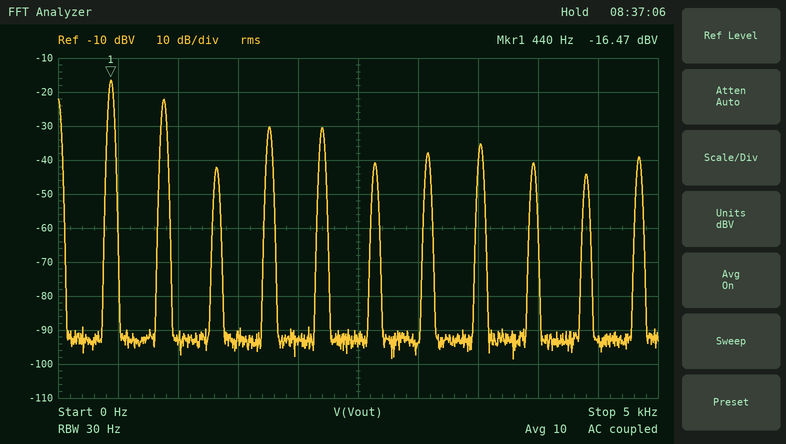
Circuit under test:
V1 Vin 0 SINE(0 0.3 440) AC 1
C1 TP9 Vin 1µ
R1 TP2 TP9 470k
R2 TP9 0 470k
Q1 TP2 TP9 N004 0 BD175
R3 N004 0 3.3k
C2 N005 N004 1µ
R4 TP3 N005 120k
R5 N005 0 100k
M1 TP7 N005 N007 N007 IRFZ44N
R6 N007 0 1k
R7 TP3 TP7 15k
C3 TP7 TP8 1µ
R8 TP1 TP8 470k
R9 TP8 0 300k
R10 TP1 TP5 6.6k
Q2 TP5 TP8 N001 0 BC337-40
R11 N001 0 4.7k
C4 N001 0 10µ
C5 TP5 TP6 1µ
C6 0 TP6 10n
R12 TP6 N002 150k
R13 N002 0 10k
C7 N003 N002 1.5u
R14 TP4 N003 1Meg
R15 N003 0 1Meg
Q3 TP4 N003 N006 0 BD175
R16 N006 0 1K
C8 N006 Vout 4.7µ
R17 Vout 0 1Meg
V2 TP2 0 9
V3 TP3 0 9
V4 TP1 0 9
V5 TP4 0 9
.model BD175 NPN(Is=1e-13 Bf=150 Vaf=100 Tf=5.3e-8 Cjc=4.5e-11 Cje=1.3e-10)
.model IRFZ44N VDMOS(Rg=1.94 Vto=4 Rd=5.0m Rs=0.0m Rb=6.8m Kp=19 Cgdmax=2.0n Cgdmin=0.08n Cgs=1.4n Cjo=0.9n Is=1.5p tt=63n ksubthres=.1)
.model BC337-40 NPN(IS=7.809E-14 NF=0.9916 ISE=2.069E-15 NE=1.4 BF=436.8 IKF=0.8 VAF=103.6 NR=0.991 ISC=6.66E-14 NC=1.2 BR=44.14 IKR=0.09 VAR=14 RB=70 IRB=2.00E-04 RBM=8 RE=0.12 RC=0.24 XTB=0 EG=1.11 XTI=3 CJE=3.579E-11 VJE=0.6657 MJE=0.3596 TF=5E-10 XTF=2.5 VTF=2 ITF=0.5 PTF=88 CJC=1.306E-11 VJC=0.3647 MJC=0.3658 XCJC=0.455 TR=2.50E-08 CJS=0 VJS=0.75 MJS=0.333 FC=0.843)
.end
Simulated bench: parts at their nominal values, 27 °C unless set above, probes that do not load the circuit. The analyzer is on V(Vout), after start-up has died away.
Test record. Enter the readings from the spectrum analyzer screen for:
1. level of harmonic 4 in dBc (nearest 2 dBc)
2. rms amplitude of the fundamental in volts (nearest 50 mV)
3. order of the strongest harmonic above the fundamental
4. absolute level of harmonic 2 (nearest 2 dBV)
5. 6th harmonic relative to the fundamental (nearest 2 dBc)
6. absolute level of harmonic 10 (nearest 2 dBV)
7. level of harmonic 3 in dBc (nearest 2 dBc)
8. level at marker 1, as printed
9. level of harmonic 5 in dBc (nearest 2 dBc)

-14 dBc
150 mV
2
-22 dBV
-24 dBc
-44 dBV
-26 dBc
-16.47 dBV
-14 dBc
